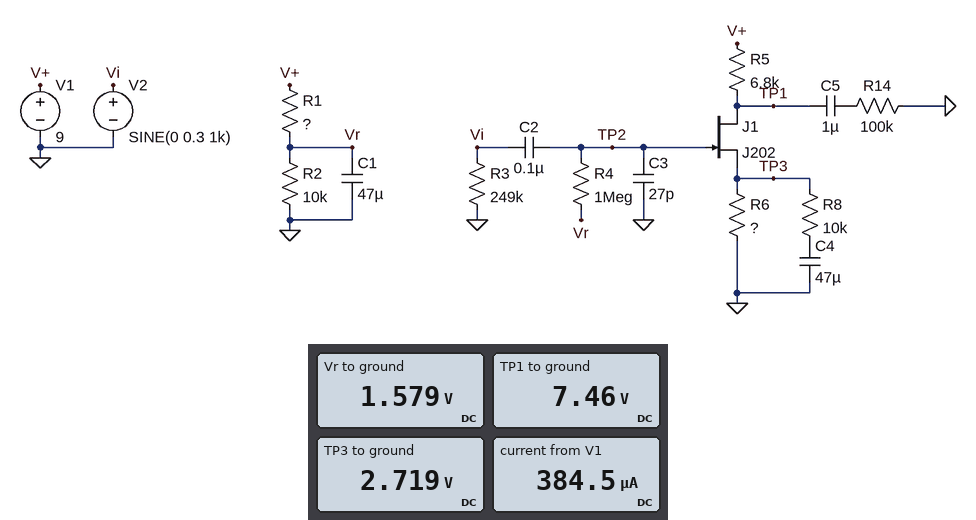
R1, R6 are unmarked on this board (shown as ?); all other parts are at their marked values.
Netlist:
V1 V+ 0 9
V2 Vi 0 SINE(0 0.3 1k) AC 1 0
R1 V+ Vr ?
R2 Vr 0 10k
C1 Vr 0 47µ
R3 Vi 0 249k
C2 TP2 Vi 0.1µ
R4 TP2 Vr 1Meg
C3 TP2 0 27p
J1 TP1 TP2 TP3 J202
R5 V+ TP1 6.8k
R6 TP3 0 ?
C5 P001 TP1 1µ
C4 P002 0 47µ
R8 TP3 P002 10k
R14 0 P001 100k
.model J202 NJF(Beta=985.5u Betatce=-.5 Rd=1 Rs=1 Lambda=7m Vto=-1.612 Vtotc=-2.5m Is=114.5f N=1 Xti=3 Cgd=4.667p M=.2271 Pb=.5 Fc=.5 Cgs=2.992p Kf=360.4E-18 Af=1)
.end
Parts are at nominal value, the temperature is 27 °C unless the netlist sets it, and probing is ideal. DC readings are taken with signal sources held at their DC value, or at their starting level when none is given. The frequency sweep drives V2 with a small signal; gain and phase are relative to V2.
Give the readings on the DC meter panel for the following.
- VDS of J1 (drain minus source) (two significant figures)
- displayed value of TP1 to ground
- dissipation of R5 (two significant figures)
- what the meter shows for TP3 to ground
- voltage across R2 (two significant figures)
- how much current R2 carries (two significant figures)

4.7 V
7.46 V
350 µW
2.719 V
1.6 V
160 µA
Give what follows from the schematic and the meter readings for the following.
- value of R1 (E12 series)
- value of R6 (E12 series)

47 kΩ
12 kΩ
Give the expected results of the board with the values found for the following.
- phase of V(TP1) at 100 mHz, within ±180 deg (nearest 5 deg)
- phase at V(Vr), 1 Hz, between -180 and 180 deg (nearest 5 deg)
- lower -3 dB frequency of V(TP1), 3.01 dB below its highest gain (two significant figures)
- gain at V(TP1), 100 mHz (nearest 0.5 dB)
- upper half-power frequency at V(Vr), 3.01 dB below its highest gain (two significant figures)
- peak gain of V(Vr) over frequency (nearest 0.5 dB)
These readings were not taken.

-80 deg
-10 deg
1.5 Hz
-28.5 dB
2.3 Hz
-55.5 dB
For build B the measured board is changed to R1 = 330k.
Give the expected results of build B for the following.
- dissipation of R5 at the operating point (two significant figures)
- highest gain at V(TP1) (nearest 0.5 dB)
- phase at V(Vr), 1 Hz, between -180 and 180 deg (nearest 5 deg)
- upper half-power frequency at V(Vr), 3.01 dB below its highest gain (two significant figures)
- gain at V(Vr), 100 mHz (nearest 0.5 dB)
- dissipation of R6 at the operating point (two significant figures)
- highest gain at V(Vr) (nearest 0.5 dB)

110 µW
-0.5 dB
-15 deg
2.2 Hz
-64.5 dB
190 µW
-55.0 dB
